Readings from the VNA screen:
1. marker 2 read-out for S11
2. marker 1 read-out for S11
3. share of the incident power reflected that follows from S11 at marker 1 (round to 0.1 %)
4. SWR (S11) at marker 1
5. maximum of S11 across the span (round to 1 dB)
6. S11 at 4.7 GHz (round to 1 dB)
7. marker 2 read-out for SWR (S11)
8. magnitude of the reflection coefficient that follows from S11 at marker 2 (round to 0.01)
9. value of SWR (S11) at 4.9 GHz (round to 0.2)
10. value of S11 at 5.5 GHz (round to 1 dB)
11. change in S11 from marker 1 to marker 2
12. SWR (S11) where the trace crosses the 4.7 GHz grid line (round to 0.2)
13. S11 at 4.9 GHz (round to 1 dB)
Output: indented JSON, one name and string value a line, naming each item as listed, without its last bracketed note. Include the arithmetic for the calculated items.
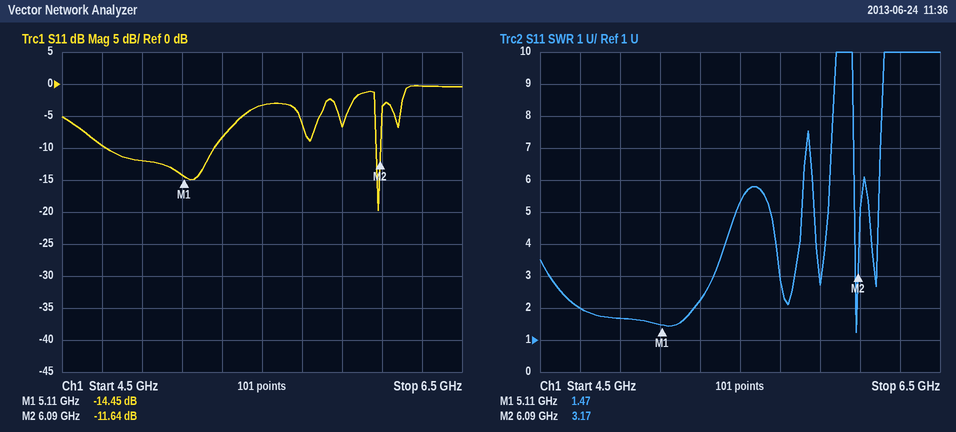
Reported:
{
  "marker 2 read-out for S11": "-11.64 dB",
  "marker 1 read-out for S11": "-14.45 dB",
  "share of the incident power reflected that follows from S11 at marker 1": "10^(-14.45/10) ≈ 3.6 %",
  "SWR (S11) at marker 1": "1.47",
  "maximum of S11 across the span": "0 dB",
  "S11 at 4.7 GHz": "-10 dB",
  "marker 2 read-out for SWR": "3.17",
  "magnitude of the reflection coefficient that follows from S11 at marker 2": "10^(-11.64/20) ≈ 0.26",
  "value of SWR (S11) at 4.9 GHz": "1.6",
  "value of S11 at 5.5 GHz": "-3 dB",
  "change in S11 from marker 1 to marker 2": "-11.64 − (-14.45) = 2.81 dB",
  "SWR (S11) where the trace crosses the 4.7 GHz grid line": "2.0",
  "S11 at 4.9 GHz": "-12 dB"
}
